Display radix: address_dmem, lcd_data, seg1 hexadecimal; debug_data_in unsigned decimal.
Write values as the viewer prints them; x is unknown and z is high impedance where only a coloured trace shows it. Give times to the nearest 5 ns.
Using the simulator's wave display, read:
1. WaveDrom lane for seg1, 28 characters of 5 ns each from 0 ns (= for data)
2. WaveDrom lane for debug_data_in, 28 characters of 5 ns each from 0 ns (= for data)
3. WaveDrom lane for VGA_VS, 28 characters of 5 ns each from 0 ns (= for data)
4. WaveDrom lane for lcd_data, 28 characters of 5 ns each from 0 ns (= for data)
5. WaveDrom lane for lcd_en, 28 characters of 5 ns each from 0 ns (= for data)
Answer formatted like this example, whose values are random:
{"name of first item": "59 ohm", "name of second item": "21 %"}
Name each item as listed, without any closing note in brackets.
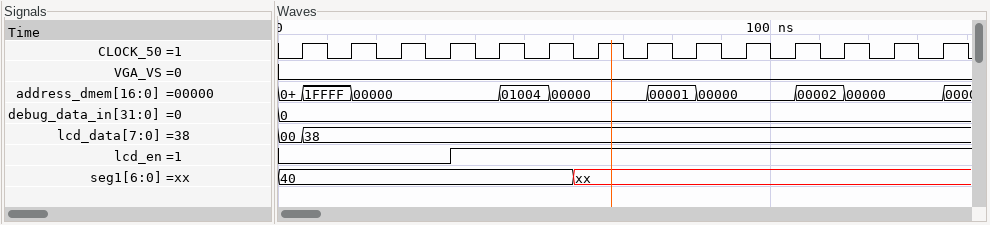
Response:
{"WaveDrom lane for seg1, 28 characters of 5 ns each from 0 ns": "{name: 'seg1', wave: '=...........x...............', data: '40'}", "WaveDrom lane for debug_data_in, 28 characters of 5 ns each from 0 ns": "{name: 'debug_data_in', wave: '=...........................', data: '0'}", "WaveDrom lane for VGA_VS, 28 characters of 5 ns each from 0 ns": "{name: 'VGA_VS', wave: '0...........................'}", "WaveDrom lane for lcd_data, 28 characters of 5 ns each from 0 ns": "{name: 'lcd_data', wave: '==..........................', data: '00 38'}", "WaveDrom lane for lcd_en, 28 characters of 5 ns each from 0 ns": "{name: 'lcd_en', wave: '0......1....................'}"}
